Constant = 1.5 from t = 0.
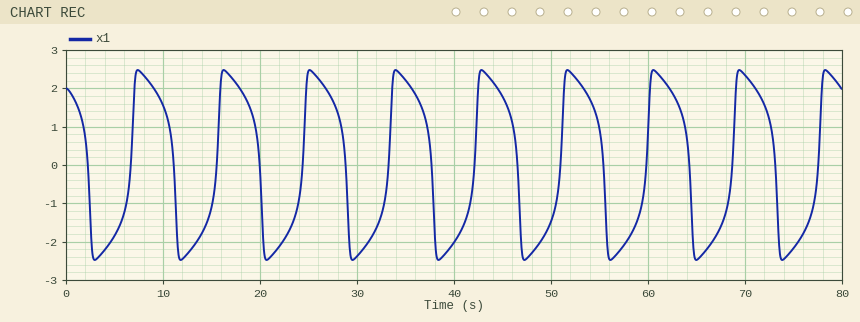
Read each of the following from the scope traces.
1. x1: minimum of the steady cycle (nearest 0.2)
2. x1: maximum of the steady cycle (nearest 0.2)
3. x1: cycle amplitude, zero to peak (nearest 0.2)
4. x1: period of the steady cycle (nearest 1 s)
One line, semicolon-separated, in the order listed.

-2.4; 2.4; 2.4; 9 s
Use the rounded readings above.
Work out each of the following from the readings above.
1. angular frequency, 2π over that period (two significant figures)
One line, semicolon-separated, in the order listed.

0.70 rad/s
